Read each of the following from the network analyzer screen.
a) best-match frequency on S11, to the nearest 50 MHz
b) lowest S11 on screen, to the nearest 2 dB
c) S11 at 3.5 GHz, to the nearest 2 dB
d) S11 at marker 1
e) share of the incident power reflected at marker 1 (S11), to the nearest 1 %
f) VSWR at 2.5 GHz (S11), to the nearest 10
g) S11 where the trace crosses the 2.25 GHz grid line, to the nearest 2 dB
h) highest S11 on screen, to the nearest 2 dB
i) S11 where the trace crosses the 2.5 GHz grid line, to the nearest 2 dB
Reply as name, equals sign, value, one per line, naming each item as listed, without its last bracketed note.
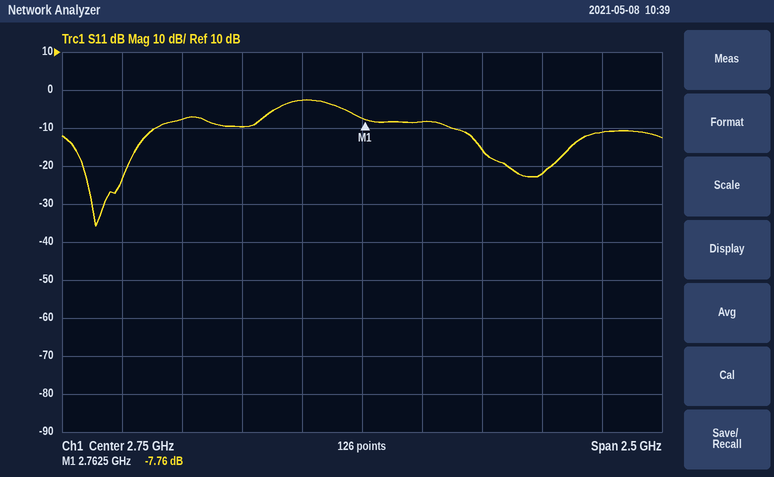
best-match frequency on S11, to the nearest 50 MHz = 1.65 GHz
lowest S11 on screen, to the nearest 2 dB = -36 dB
S11 at 3.5 GHz, to the nearest 2 dB = -22 dB
S11 at marker 1 = -7.76 dB
share of the incident power reflected at marker 1 (S11), to the nearest 1 % = 17 %
VSWR at 2.5 GHz (S11), to the nearest 10 = 10
S11 where the trace crosses the 2.25 GHz grid line, to the nearest 2 dB = -10 dB
highest S11 on screen, to the nearest 2 dB = -2 dB
S11 where the trace crosses the 2.5 GHz grid line, to the nearest 2 dB = -2 dB
